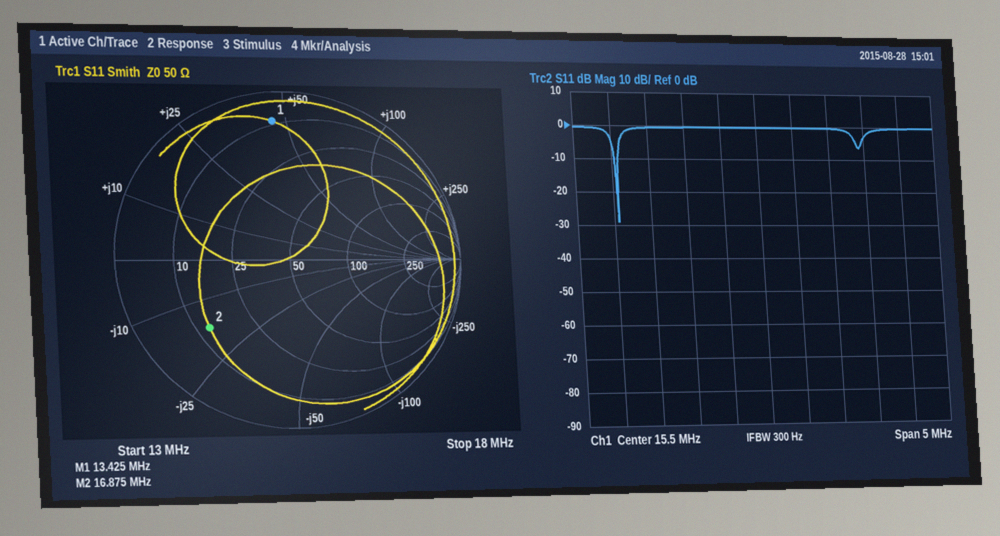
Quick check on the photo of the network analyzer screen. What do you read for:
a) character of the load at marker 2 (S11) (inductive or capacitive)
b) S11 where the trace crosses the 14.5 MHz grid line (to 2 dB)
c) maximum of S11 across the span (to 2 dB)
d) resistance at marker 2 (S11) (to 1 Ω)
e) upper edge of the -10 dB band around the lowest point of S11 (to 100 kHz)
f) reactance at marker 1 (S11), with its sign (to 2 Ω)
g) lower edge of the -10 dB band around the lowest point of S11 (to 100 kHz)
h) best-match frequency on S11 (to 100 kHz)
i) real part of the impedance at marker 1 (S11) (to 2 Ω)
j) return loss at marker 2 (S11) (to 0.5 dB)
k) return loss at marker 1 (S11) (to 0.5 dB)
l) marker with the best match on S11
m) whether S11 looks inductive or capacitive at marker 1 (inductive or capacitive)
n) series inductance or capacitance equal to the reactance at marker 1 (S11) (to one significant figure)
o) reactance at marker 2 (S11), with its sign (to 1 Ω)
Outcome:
capacitive
0 dB
0 dB
13 Ω
13.6 MHz
+46 Ω
13.5 MHz
13.6 MHz
8 Ω
4.0 dB
1.5 dB
marker 2
inductive
500 nH
-17 Ω
